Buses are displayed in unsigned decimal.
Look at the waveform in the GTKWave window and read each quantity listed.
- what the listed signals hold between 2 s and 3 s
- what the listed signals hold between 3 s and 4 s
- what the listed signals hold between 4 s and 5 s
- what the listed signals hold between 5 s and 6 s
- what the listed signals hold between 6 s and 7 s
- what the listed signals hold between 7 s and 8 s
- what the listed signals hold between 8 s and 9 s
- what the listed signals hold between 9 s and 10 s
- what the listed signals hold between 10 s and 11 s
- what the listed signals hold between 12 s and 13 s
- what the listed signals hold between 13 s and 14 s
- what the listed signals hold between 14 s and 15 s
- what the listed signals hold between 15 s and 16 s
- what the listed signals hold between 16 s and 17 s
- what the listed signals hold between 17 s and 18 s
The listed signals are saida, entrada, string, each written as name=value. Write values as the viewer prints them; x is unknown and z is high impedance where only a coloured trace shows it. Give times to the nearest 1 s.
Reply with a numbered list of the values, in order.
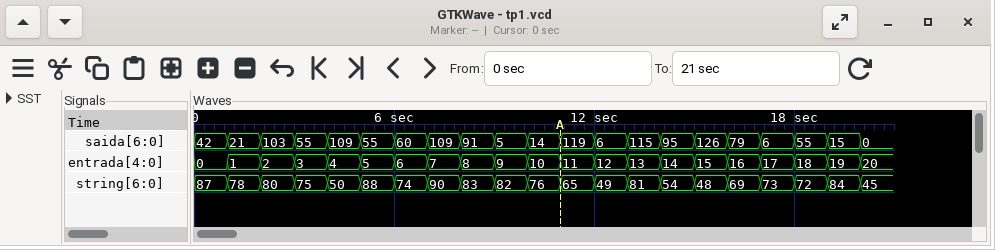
1. saida=103, entrada=2, string=80
2. saida=55, entrada=3, string=75
3. saida=109, entrada=4, string=50
4. saida=55, entrada=5, string=88
5. saida=60, entrada=6, string=74
6. saida=109, entrada=7, string=90
7. saida=91, entrada=8, string=83
8. saida=5, entrada=9, string=82
9. saida=14, entrada=10, string=76
10. saida=6, entrada=12, string=49
11. saida=115, entrada=13, string=81
12. saida=95, entrada=14, string=54
13. saida=126, entrada=15, string=48
14. saida=79, entrada=16, string=69
15. saida=6, entrada=17, string=73
